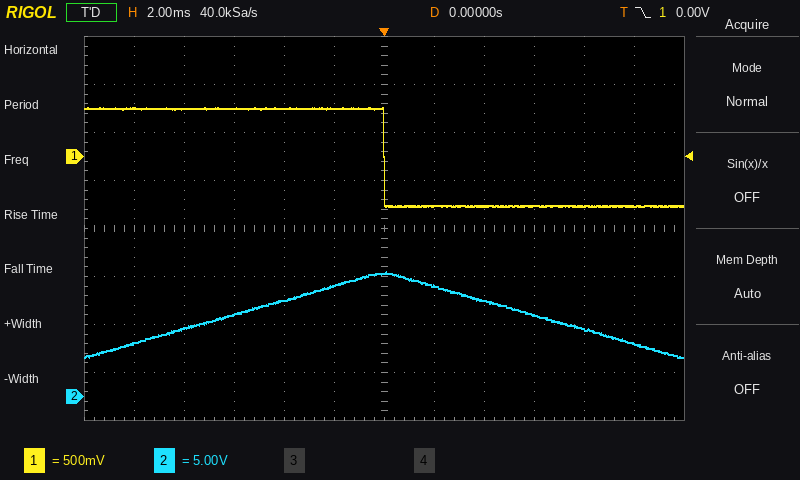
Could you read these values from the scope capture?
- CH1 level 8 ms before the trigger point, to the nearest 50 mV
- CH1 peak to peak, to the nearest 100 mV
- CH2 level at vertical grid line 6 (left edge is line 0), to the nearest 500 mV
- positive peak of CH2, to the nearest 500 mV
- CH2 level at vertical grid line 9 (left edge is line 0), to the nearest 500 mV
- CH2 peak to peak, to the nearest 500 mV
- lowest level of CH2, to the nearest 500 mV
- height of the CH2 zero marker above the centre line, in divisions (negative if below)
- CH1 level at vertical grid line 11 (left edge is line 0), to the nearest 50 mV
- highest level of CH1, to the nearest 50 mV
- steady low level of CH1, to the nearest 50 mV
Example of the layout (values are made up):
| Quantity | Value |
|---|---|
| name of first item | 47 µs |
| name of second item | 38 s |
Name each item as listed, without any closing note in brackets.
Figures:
| Quantity | Value |
|---|---|
| CH1 level 8 ms before the trigger point, to the nearest 50 mV | 500 mV |
| CH1 peak to peak, to the nearest 100 mV | 1.00 V |
| CH2 level at vertical grid line 6 (left edge is line 0), to the nearest 500 mV | 13.0 V |
| positive peak of CH2, to the nearest 500 mV | 13.0 V |
| CH2 level at vertical grid line 9 (left edge is line 0), to the nearest 500 mV | 8.5 V |
| CH2 peak to peak, to the nearest 500 mV | 9.0 V |
| lowest level of CH2, to the nearest 500 mV | 4.0 V |
| height of the CH2 zero marker above the centre line, in divisions | -3.5 div |
| CH1 level at vertical grid line 11 (left edge is line 0), to the nearest 50 mV | -500 mV |
| highest level of CH1, to the nearest 50 mV | 500 mV |
| steady low level of CH1, to the nearest 50 mV | -500 mV |
